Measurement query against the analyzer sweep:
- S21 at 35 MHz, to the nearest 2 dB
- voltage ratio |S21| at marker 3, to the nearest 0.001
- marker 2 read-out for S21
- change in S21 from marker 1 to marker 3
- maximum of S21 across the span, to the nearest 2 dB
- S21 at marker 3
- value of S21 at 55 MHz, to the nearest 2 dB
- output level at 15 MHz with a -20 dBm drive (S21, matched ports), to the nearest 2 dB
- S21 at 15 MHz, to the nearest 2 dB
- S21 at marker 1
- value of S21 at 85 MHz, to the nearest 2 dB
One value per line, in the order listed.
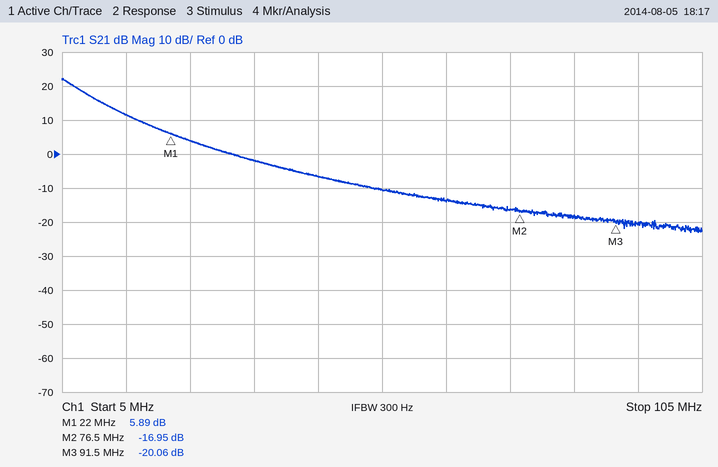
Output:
-2 dB
0.099
-16.95 dB
-25.95 dB
22 dB
-20.06 dB
-10 dB
-8 dBm
12 dB
5.89 dB
-18 dB
